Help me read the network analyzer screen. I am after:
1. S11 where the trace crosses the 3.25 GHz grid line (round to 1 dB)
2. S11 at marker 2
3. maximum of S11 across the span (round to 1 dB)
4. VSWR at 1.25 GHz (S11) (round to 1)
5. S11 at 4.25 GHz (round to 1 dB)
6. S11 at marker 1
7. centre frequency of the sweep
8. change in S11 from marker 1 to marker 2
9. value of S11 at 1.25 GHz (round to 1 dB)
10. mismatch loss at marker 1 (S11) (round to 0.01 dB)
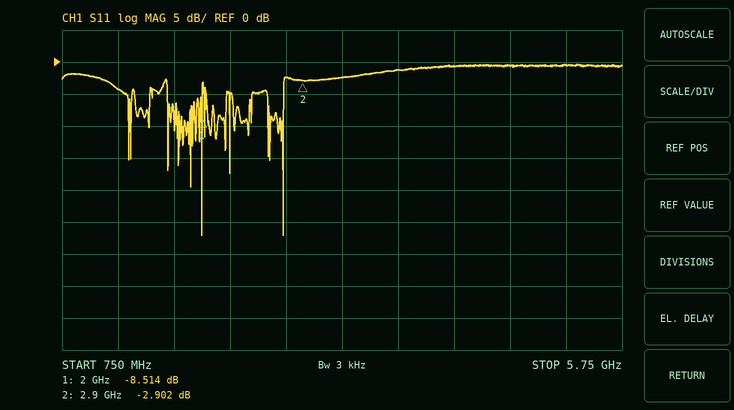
-2 dB
-2.902 dB
0 dB
4
-1 dB
-8.514 dB
3.25 GHz
5.612 dB
-4 dB
0.66 dB
